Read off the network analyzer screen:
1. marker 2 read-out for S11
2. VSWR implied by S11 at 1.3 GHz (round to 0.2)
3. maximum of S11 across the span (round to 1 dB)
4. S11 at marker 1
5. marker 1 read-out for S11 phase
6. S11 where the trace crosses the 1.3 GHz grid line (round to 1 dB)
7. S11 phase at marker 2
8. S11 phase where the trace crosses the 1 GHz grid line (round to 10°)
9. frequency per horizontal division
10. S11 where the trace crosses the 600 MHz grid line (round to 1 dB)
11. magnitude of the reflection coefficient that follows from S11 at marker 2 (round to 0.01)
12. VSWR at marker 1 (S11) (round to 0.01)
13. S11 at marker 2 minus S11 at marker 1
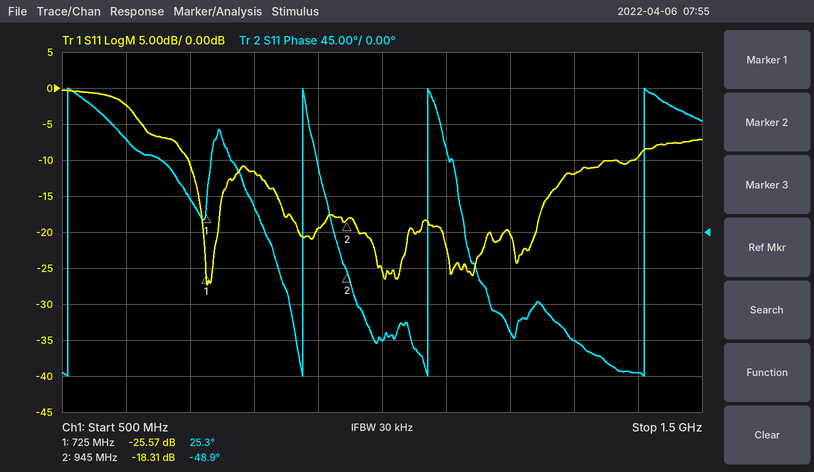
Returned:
-18.31 dB
1.6
0 dB
-25.57 dB
25.3°
-12 dB
-48.9°
-140°
100 MHz
-2 dB
0.12
1.11
7.26 dB
